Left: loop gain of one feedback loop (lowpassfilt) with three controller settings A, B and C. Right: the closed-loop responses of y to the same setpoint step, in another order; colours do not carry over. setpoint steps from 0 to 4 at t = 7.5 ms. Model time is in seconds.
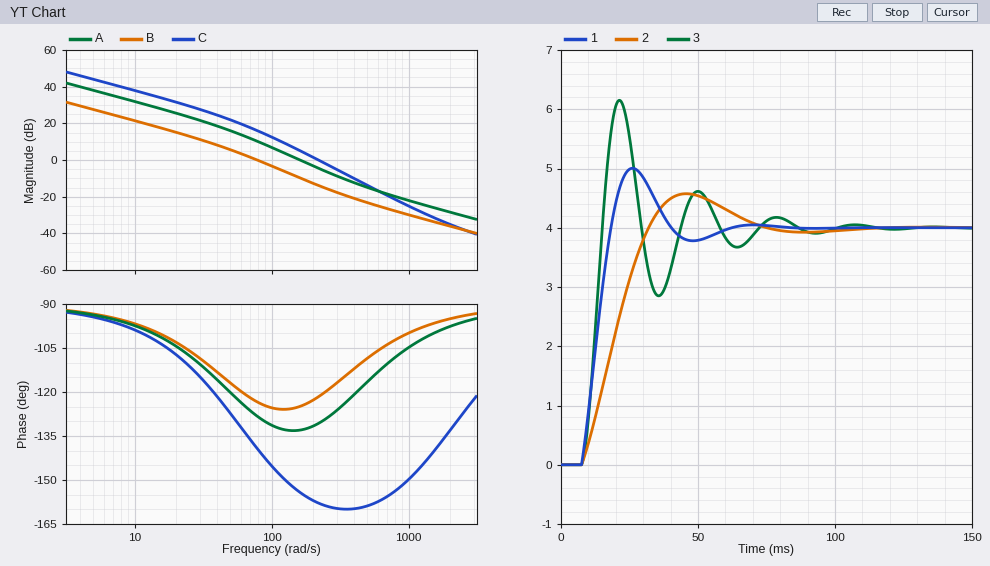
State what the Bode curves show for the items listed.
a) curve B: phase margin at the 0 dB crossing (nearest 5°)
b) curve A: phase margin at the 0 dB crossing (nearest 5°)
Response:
55°
45°
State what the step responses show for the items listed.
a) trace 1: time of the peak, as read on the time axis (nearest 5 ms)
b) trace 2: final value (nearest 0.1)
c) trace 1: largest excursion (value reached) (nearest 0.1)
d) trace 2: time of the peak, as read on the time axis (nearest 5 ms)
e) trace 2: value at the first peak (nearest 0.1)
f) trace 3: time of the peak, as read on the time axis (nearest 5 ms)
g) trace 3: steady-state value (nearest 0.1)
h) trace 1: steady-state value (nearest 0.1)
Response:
25 ms
4.0
5.0
45 ms
4.6
20 ms
4.0
4.0
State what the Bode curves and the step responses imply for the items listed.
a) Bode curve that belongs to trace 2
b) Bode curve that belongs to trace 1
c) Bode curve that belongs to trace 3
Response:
B
A
C
